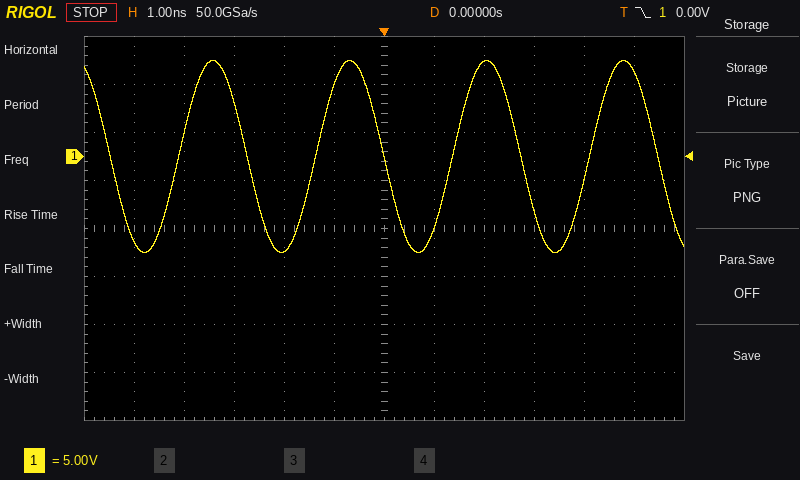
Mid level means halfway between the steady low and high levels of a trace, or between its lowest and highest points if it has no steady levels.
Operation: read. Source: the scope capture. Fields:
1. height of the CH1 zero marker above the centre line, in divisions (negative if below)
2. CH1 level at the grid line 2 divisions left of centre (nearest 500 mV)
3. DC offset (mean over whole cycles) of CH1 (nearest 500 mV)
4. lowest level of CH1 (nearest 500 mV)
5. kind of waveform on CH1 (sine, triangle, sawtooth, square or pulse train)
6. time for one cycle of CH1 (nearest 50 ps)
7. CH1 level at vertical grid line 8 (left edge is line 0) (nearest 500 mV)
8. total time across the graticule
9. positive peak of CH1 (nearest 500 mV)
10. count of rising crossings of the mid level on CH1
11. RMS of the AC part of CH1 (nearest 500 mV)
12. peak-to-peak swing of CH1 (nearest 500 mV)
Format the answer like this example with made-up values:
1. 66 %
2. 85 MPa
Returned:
1. +1.5 div
2. -10.0 V
3. 0.0 V
4. -10.0 V
5. sine
6. 2.75 ns
7. 10.0 V
8. 12 ns
9. 10.0 V
10. 4
11. 7.0 V
12. 20.0 V
